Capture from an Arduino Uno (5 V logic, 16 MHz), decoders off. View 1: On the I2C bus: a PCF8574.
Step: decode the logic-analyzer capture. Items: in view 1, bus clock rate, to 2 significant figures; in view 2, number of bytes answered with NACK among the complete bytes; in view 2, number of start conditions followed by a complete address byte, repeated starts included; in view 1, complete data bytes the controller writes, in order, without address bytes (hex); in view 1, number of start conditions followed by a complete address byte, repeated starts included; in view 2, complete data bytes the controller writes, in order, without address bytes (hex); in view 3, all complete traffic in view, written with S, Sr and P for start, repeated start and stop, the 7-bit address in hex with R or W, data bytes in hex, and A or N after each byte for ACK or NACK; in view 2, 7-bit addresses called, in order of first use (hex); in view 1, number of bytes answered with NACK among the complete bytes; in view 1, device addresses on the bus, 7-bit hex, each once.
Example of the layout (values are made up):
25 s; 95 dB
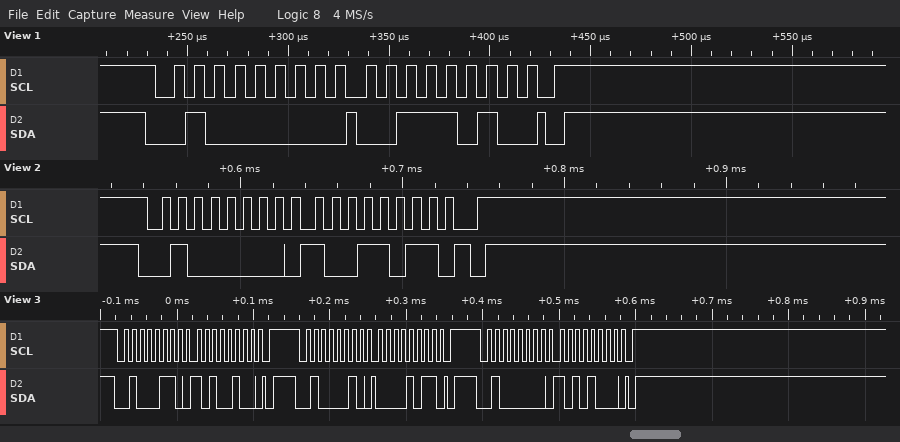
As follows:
100 kHz; 0; 1; 3A; 1; 9B; S 23W A A4 A P S 21W A 0B A P S 20W A A8 A P; 0x20; 0; 0x20
